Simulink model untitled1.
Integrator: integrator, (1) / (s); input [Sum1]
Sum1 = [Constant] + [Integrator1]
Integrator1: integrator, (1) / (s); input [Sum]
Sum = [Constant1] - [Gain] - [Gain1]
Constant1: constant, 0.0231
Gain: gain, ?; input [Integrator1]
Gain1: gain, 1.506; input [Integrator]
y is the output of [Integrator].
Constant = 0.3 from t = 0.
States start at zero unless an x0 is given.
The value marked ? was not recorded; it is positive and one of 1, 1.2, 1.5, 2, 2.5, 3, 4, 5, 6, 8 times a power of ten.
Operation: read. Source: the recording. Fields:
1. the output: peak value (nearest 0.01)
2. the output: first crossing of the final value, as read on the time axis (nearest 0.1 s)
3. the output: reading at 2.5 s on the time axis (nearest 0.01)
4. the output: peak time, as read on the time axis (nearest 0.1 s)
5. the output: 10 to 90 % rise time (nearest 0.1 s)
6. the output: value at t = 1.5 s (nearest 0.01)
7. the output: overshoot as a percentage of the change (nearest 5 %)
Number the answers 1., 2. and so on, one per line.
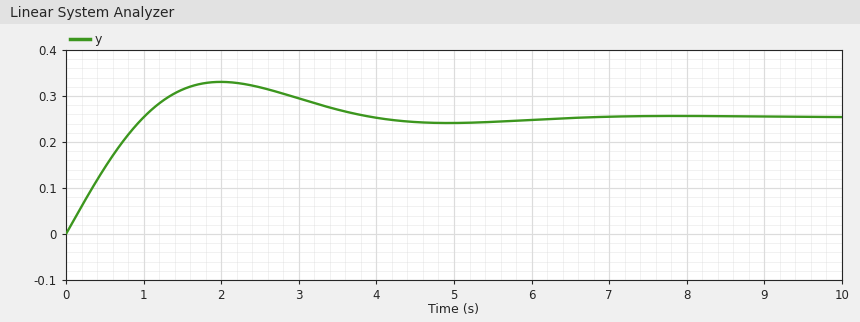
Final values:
1. 0.33
2. 1.0 s
3. 0.32
4. 2.0 s
5. 0.8 s
6. 0.31
7. 30 %
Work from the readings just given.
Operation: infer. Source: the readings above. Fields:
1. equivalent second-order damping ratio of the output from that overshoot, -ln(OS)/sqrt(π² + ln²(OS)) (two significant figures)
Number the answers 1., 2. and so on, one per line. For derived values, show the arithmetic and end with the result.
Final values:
1. ln(0.3) = -1.204; 1.204 / sqrt(9.870 + 1.450) = 0.36
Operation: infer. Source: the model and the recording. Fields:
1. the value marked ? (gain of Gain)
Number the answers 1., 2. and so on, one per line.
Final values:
1. 1.2
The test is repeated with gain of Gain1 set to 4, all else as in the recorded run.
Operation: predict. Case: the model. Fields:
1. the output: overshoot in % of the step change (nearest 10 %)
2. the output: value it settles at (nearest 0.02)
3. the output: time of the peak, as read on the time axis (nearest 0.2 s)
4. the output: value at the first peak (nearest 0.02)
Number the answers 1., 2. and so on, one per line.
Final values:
1. 90 %
2. 0.10
3. 1.0 s
4. 0.18
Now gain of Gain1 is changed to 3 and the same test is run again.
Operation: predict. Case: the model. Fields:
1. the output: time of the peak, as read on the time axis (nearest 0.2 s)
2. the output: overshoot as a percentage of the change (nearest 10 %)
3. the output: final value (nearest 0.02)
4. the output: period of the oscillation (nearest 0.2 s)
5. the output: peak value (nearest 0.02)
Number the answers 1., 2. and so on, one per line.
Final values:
1. 1.2 s
2. 70 %
3. 0.12
4. 3.8 s
5. 0.22
